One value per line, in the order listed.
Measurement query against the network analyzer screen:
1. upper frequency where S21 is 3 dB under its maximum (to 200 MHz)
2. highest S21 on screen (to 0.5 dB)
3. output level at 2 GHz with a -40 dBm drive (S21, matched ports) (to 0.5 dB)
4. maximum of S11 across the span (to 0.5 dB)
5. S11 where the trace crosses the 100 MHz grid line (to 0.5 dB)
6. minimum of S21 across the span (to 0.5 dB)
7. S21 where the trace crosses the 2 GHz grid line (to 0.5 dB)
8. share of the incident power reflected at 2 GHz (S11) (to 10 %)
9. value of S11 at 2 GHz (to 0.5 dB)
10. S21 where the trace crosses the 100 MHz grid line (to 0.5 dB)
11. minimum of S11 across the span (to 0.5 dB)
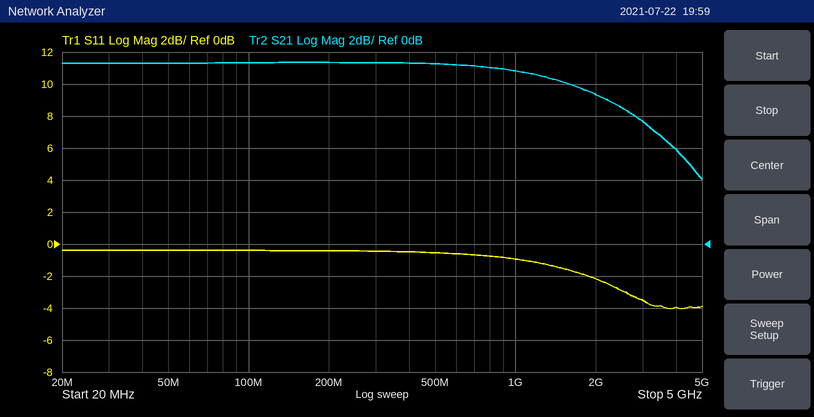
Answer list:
2.6 GHz
11.5 dB
-30.5 dBm
-0.5 dB
-0.5 dB
4.0 dB
9.5 dB
60 %
-2.0 dB
11.5 dB
-4.0 dB
